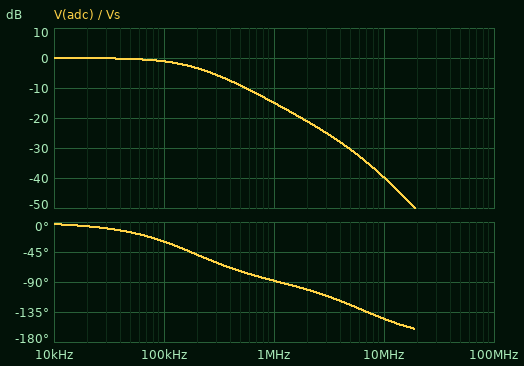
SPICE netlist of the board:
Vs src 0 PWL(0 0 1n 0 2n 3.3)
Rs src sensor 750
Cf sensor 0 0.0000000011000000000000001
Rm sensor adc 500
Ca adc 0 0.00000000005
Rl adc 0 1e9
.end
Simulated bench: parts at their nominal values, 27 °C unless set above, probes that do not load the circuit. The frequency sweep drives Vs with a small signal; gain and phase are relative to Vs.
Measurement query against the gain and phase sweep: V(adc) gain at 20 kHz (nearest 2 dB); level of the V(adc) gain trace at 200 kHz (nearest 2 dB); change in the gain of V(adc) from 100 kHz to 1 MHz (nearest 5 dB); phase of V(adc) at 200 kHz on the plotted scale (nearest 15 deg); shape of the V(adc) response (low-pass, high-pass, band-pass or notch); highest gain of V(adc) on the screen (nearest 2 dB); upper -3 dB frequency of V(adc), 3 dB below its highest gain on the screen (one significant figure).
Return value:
0 dB
-4 dB
-15 dB
-45 deg
low-pass
0 dB
200 kHz
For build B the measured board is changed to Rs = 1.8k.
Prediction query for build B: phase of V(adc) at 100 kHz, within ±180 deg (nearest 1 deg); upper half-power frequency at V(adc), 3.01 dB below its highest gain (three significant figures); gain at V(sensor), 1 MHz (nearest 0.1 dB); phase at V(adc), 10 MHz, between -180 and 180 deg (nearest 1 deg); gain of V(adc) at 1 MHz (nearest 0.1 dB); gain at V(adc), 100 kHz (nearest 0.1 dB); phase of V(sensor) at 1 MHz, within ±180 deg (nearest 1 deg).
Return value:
-53 deg
76.8 kHz
-22.3 dB
-146 deg
-22.4 dB
-4.3 dB
-85 deg
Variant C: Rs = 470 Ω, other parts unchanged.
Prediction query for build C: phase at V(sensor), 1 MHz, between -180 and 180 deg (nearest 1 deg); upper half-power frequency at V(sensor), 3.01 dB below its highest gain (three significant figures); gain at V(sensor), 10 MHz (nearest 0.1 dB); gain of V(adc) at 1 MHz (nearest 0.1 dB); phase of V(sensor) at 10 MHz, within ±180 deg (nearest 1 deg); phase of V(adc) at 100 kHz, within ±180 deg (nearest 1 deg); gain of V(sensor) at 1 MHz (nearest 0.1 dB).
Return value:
-73 deg
294 kHz
-30.4 dB
-11.1 dB
-87 deg
-20 deg
-11.0 dB
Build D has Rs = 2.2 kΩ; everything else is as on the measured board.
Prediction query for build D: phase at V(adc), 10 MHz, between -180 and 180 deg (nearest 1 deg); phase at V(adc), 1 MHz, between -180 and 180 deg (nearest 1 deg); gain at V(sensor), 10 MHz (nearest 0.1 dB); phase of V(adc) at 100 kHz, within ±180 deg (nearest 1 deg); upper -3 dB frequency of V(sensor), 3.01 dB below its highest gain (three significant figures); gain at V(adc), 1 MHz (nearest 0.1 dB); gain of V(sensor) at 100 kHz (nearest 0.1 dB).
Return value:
-146 deg
-95 deg
-43.8 dB
-59 deg
62.9 kHz
-24.1 dB
-5.5 dB
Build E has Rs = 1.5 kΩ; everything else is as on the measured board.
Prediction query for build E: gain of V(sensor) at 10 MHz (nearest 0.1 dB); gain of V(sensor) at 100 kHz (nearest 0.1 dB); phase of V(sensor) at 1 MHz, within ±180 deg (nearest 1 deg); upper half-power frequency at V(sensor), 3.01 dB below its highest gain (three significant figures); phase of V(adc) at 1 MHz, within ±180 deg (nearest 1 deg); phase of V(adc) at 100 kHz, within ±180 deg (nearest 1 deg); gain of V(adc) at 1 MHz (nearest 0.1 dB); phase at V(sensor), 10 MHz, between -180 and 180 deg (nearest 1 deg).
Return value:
-40.4 dB
-3.4 dB
-84 deg
92.2 kHz
-93 deg
-48 deg
-20.8 dB
-88 deg
